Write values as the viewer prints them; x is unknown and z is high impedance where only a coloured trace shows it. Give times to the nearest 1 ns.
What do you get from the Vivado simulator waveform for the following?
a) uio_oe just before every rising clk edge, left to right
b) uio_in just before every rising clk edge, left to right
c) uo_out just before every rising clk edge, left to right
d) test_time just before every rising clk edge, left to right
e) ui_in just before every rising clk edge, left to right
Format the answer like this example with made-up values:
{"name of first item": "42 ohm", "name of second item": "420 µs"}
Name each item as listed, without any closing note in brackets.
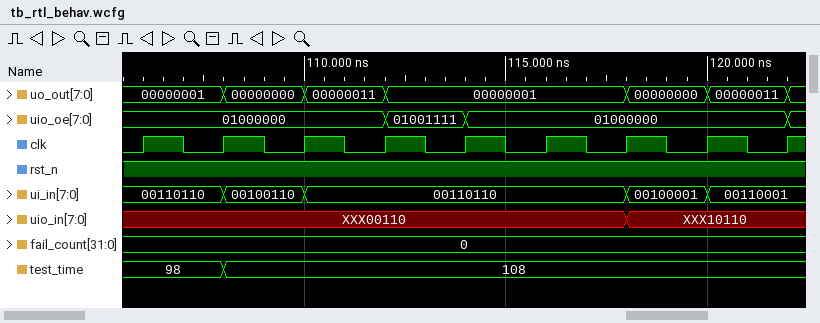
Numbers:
{"uio_oe just before every rising clk edge, left to right": "01000000, 01000000, 01000000, 01000000, 01001111, 01000000, 01000000, 01000000, 01000000", "uio_in just before every rising clk edge, left to right": "XXX00110, XXX00110, XXX00110, XXX00110, XXX00110, XXX00110, XXX00110, XXX10110, XXX10110", "uo_out just before every rising clk edge, left to right": "00000001, 00000001, 00000000, 00000011, 00000001, 00000001, 00000001, 00000000, 00000011", "test_time just before every rising clk edge, left to right": "98, 98, 108, 108, 108, 108, 108, 108, 108", "ui_in just before every rising clk edge, left to right": "00110110, 00110110, 00100110, 00110110, 00110110, 00110110, 00110110, 00100001, 00110001"}
